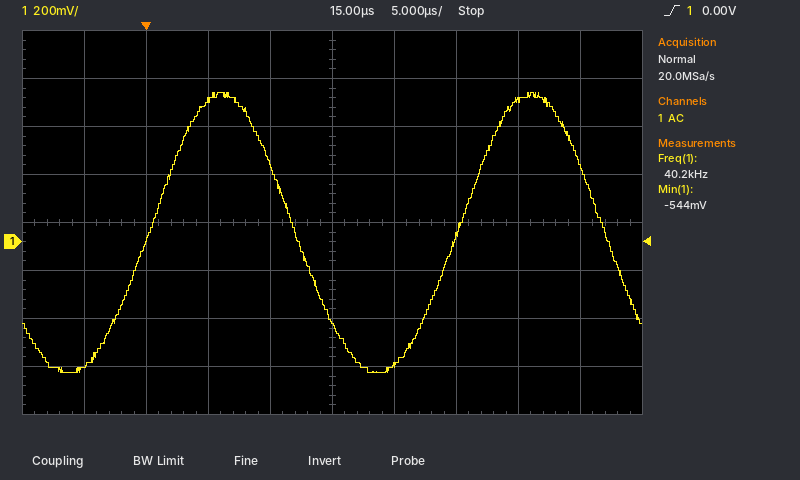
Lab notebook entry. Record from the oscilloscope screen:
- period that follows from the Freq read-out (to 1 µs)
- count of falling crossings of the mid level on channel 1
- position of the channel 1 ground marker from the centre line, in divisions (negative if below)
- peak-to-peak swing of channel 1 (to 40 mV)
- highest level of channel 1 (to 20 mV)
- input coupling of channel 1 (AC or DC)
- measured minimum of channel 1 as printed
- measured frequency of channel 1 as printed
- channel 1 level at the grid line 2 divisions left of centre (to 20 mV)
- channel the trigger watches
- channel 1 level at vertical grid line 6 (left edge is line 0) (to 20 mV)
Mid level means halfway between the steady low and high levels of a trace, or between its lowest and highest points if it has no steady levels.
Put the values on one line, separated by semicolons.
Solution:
25 µs; 2; -0.4 div; 1.16 V; 620 mV; AC; -544 mV; 40.2 kHz; 580 mV; channel 1; -520 mV
